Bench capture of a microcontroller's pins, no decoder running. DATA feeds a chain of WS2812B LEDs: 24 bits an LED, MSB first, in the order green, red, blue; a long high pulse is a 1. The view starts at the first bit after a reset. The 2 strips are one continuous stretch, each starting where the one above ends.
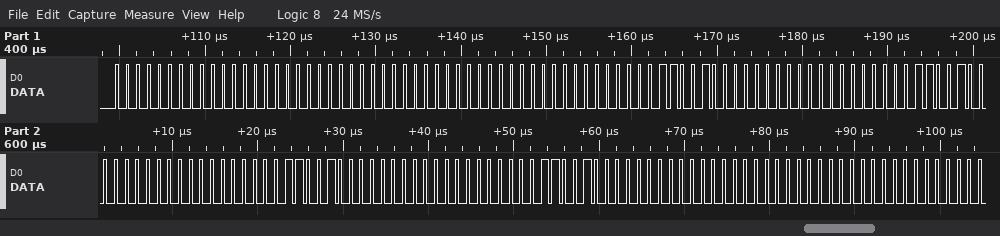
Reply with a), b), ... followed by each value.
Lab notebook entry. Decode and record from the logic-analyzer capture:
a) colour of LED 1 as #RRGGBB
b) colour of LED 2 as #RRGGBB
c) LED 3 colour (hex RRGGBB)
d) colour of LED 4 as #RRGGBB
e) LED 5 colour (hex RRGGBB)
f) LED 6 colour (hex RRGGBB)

a) #000000
b) #000000
c) #001900
d) #001900
e) #001900
f) #001900
